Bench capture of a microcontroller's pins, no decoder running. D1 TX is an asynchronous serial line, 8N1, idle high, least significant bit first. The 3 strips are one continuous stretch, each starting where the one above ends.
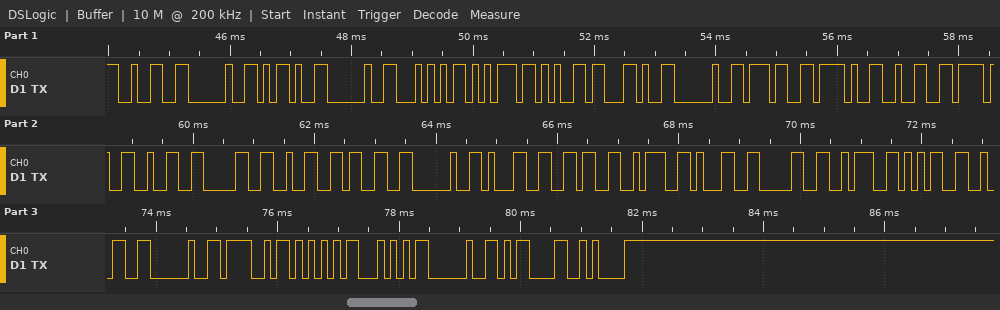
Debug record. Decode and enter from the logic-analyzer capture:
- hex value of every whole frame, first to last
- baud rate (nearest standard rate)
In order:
0x32 0x20 0x2D 0x20 0x54 0x75 0x65 0x2C 0x20 0x37 0x2F 0x32 0x2F 0x32 0x30 0x32 0x33 0x20 0x31 0x36 0x3A 0x31 0x30 0x3A 0x35 0x32 0x20 0x4F 0x55 0x54 0x20 0x0D 0x0A
9600 baud
